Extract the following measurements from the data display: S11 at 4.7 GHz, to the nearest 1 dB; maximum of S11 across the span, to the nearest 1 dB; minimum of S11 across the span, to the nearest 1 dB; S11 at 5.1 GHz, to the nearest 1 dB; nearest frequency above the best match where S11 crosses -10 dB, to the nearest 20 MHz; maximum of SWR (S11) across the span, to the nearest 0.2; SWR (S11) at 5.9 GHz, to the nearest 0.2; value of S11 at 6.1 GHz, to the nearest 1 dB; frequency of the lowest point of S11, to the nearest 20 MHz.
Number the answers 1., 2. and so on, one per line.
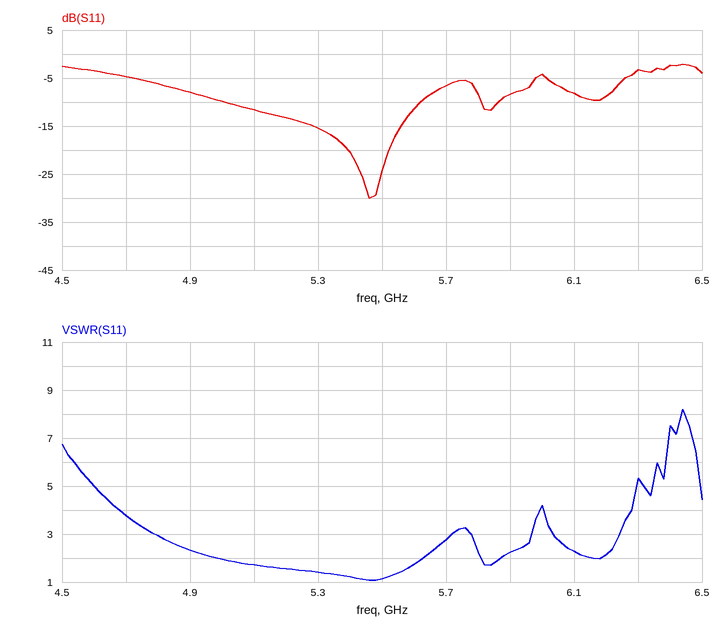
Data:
1. -5 dB
2. -2 dB
3. -30 dB
4. -12 dB
5. 5.62 GHz
6. 8.2
7. 2.2
8. -8 dB
9. 5.46 GHz
